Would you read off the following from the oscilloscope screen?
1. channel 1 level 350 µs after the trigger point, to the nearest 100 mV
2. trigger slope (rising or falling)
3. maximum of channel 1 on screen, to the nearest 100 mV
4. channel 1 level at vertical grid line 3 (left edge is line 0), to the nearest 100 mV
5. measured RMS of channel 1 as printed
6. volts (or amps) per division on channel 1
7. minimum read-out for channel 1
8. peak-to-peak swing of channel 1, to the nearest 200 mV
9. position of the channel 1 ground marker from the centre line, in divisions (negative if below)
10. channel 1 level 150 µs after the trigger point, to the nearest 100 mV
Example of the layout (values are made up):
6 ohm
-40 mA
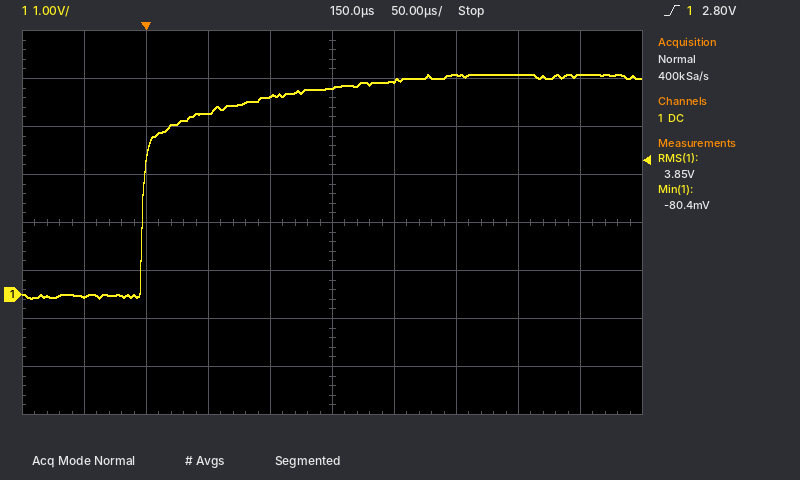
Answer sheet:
4.6 V
rising
4.6 V
3.8 V
3.85 V
1 V
-80.4 mV
4.6 V
-1.5 div
4.3 V
